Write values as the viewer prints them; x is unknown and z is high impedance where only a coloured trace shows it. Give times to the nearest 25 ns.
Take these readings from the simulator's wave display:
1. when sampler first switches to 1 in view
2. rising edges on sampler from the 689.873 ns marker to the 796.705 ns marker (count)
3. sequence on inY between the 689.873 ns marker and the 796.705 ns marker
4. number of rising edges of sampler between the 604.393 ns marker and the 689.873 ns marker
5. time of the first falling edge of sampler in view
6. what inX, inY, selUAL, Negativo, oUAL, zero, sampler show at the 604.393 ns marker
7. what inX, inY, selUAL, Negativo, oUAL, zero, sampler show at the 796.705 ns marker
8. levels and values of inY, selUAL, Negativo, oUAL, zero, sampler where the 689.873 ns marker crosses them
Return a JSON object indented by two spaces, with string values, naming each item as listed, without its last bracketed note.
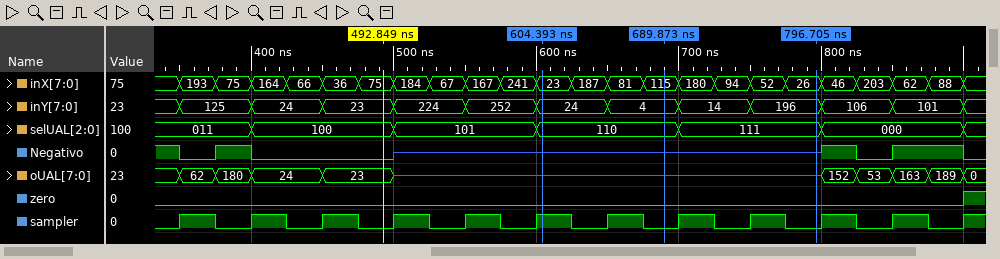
{
  "when sampler first switches to 1 in view": "350 ns",
  "rising edges on sampler from the 689.873 ns marker to the 796.705 ns marker": "2",
  "sequence on inY between the 689.873 ns marker and the 796.705 ns marker": "4, 14, 196",
  "number of rising edges of sampler between the 604.393 ns marker and the 689.873 ns marker": "1",
  "time of the first falling edge of sampler in view": "375 ns",
  "what inX, inY, selUAL, Negativo, oUAL, zero, sampler show at the 604.393 ns marker": "inX=23, inY=24, selUAL=110, Negativo=z, oUAL=z, zero=0, sampler=1",
  "what inX, inY, selUAL, Negativo, oUAL, zero, sampler show at the 796.705 ns marker": "inX=26, inY=196, selUAL=111, Negativo=z, oUAL=z, zero=0, sampler=0",
  "levels and values of inY, selUAL, Negativo, oUAL, zero, sampler where the 689.873 ns marker crosses them": "inY=4, selUAL=110, Negativo=z, oUAL=z, zero=0, sampler=0"
}
